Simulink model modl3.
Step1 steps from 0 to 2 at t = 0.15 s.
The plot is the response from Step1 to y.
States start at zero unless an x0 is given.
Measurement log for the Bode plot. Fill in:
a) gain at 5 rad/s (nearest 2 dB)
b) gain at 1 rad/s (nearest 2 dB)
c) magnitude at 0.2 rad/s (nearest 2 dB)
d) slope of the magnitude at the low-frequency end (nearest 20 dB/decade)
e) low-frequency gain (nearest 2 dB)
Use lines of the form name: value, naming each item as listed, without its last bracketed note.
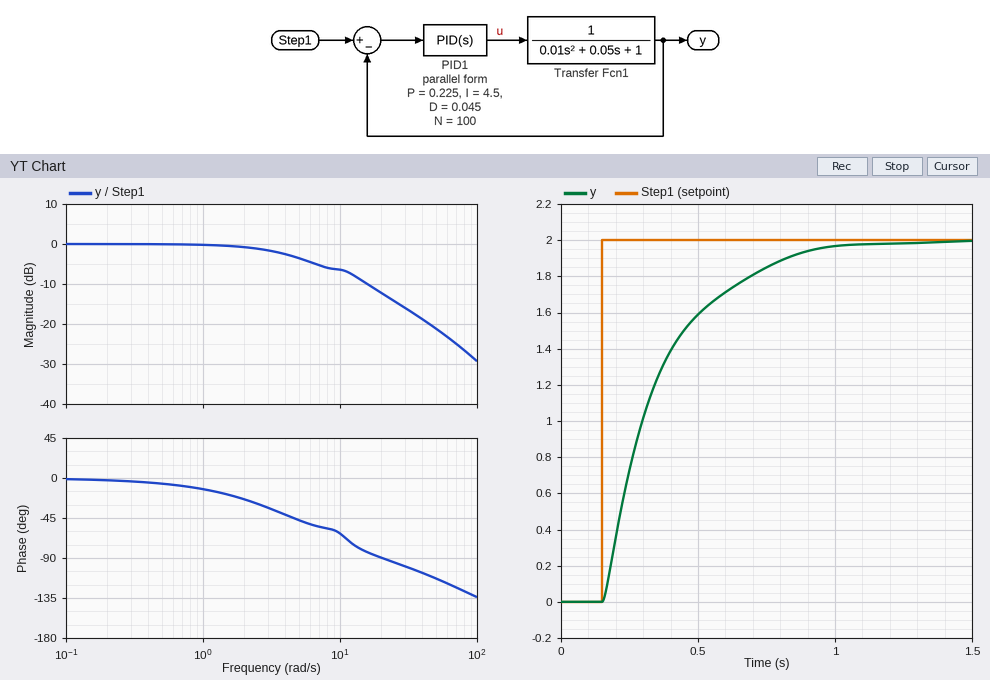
gain at 5 rad/s: -4 dB
gain at 1 rad/s: 0 dB
magnitude at 0.2 rad/s: 0 dB
slope of the magnitude at the low-frequency end: 0 dB/decade
low-frequency gain: 0 dB
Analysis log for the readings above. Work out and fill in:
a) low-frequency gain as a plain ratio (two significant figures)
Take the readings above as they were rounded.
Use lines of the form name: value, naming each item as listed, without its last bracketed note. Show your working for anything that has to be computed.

low-frequency gain as a plain ratio: 10^(0 / 20) = 1.0
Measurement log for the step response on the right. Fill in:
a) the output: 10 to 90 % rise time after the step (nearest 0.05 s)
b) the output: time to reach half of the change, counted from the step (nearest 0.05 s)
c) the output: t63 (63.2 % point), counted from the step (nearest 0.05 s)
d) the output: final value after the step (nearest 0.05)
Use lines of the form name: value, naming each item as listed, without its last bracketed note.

the output: 10 to 90 % rise time after the step: 0.50 s
the output: time to reach half of the change, counted from the step: 0.15 s
the output: t63 (63.2 % point), counted from the step: 0.20 s
the output: final value after the step: 2.00
